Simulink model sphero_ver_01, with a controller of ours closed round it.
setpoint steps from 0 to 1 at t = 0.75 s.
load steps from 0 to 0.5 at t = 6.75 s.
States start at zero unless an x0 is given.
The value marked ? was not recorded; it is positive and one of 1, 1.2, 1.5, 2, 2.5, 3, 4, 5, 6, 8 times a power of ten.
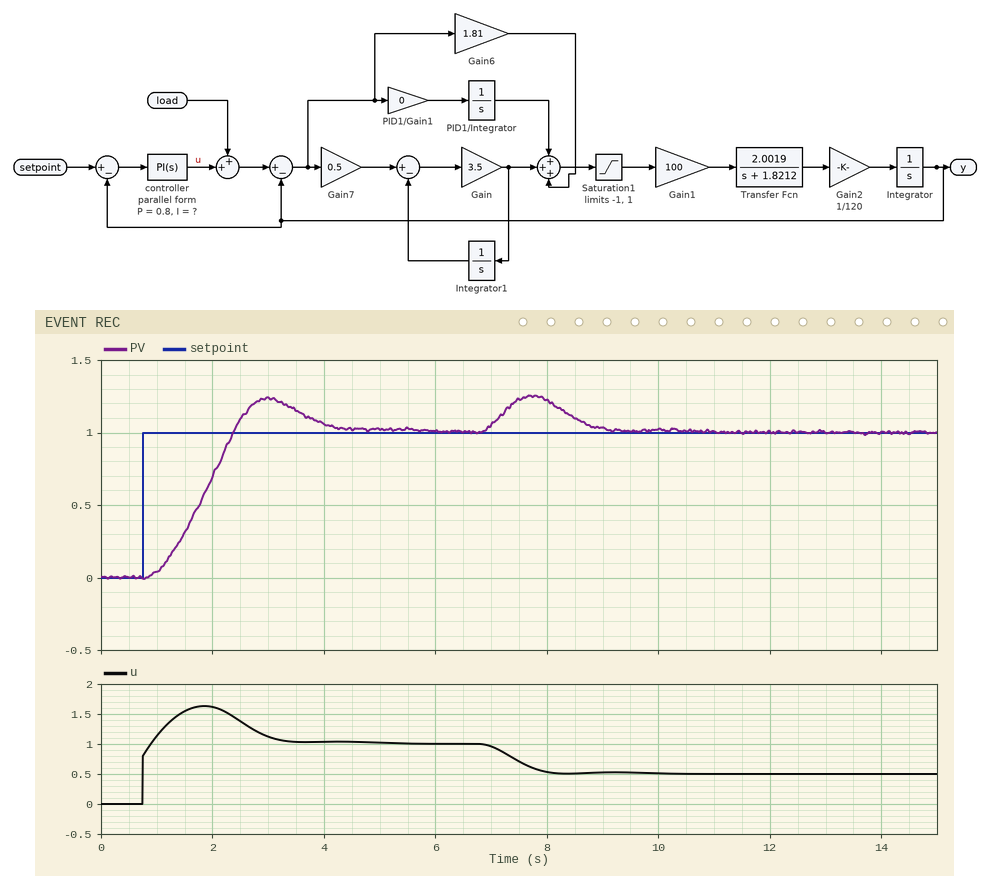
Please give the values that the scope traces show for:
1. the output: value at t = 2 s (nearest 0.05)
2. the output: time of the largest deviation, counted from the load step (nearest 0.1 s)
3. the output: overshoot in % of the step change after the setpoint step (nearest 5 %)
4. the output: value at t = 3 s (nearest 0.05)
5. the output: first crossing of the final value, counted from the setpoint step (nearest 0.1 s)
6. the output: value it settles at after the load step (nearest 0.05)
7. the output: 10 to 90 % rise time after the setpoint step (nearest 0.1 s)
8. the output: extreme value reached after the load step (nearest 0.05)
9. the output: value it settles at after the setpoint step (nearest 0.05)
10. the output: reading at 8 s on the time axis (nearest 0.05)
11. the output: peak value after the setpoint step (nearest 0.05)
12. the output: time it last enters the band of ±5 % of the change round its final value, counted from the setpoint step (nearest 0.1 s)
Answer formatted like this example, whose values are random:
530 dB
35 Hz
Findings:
0.70
1.0 s
25 %
1.25
1.6 s
1.00
1.1 s
1.25
1.00
1.20
1.25
3.3 s
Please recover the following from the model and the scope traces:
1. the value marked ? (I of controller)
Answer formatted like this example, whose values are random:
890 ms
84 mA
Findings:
1.5
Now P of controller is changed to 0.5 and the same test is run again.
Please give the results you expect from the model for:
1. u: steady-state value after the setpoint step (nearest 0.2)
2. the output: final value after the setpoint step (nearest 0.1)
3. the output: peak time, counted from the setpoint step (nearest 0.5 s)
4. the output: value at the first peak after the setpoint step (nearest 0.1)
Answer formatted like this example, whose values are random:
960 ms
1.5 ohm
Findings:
1.0
1.0
2.5 s
1.3
